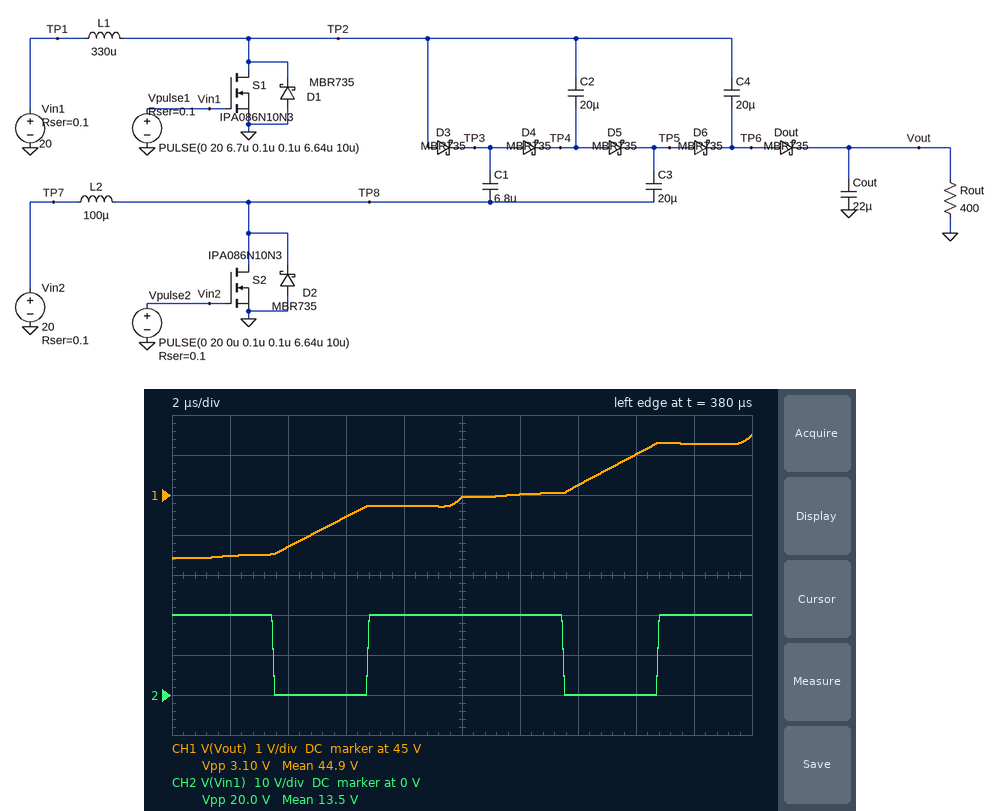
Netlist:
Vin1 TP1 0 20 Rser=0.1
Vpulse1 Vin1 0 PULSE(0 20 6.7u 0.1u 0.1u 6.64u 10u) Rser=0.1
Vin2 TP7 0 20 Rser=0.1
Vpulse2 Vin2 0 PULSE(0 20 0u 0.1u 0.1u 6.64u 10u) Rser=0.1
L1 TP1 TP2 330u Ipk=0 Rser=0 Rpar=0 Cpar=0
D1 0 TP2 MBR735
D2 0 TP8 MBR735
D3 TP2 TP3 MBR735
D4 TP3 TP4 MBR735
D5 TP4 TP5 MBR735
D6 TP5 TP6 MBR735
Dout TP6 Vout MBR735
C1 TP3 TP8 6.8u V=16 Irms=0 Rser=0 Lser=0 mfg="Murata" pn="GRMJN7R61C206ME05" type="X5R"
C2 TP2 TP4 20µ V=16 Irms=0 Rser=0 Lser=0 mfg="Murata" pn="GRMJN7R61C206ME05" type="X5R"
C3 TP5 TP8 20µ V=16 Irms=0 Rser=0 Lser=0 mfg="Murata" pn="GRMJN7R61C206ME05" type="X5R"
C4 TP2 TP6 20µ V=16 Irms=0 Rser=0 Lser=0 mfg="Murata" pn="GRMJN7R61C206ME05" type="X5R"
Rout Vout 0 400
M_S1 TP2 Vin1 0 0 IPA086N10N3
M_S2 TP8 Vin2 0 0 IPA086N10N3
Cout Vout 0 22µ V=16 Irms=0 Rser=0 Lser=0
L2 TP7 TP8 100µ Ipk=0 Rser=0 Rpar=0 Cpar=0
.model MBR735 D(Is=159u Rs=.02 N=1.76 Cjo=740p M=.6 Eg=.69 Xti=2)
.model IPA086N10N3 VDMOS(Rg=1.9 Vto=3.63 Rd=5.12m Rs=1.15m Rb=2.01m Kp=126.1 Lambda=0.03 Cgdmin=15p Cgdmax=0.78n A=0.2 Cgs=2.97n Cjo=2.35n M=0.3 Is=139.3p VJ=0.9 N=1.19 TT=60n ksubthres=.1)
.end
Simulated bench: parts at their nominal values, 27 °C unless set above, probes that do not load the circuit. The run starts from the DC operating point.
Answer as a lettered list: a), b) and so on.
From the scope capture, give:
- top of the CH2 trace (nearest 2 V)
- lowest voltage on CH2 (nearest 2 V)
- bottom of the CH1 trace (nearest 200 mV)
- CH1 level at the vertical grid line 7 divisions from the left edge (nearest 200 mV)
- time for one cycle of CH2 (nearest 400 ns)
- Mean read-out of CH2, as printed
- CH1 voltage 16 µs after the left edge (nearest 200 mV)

a) 20 V
b) 0 V
c) 43.4 V
d) 45.2 V
e) 10.0 µs
f) 13.5 V
g) 46.0 V
